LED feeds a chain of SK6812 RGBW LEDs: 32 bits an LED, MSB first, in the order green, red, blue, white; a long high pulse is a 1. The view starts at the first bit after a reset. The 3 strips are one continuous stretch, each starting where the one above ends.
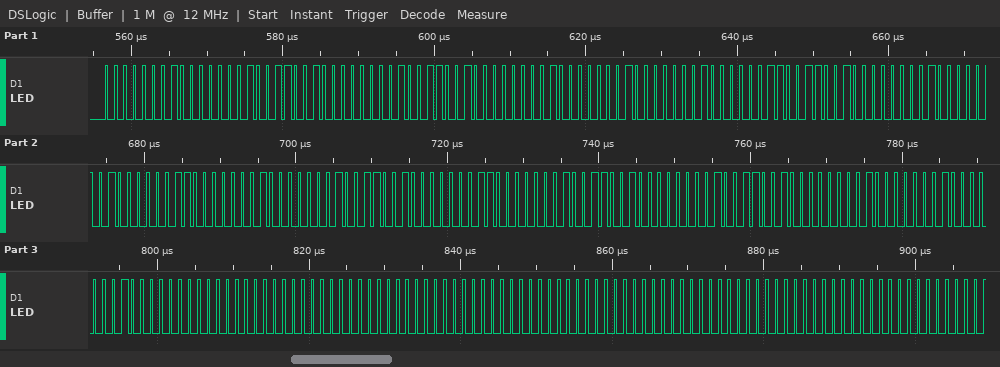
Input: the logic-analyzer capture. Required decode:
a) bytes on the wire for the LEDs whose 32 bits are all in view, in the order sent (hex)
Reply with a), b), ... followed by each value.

a) 01 01 32 01 32 01 01 01 03 32 01 01 03 01 01 32 03 01 32 01 32 01 01 01 00 00 00 00 00 00 00 00
